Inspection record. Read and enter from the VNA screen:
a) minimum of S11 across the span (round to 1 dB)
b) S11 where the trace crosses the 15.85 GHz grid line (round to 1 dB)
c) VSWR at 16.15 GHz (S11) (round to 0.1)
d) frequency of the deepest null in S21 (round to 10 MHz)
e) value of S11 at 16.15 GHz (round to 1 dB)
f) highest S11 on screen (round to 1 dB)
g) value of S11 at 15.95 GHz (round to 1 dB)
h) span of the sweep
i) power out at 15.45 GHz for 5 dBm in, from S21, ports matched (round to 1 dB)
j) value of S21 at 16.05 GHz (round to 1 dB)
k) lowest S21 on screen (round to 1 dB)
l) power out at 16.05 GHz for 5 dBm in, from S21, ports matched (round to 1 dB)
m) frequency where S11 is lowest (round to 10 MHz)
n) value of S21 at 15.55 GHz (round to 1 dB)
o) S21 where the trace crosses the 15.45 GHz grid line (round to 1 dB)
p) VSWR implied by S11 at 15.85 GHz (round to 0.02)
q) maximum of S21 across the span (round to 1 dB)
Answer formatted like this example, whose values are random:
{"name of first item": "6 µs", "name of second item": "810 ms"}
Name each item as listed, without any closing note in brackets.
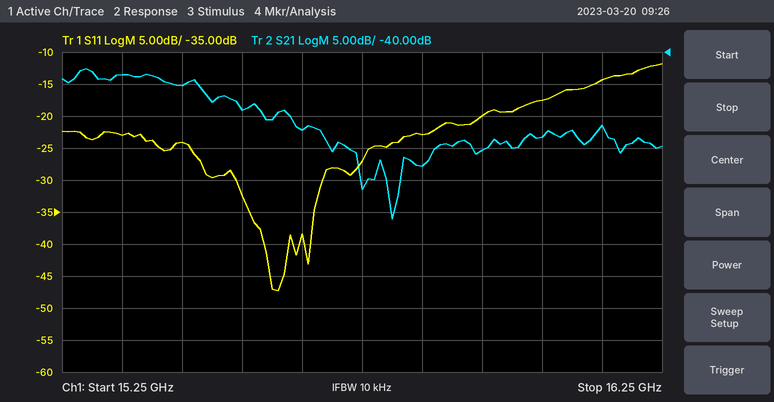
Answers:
{"minimum of S11 across the span": "-47 dB", "S11 where the trace crosses the 15.85 GHz grid line": "-23 dB", "VSWR at 16.15 GHz (S11)": "1.5", "frequency of the deepest null in S21": "15.80 GHz", "value of S11 at 16.15 GHz": "-14 dB", "highest S11 on screen": "-12 dB", "value of S11 at 15.95 GHz": "-20 dB", "span of the sweep": "1 GHz", "power out at 15.45 GHz for 5 dBm in, from S21, ports matched": "-40 dBm", "value of S21 at 16.05 GHz": "-53 dB", "lowest S21 on screen": "-66 dB", "power out at 16.05 GHz for 5 dBm in, from S21, ports matched": "-48 dBm", "frequency where S11 is lowest": "15.61 GHz", "value of S21 at 15.55 GHz": "-49 dB", "S21 where the trace crosses the 15.45 GHz grid line": "-45 dB", "VSWR implied by S11 at 15.85 GHz": "1.16", "maximum of S21 across the span": "-43 dB"}
